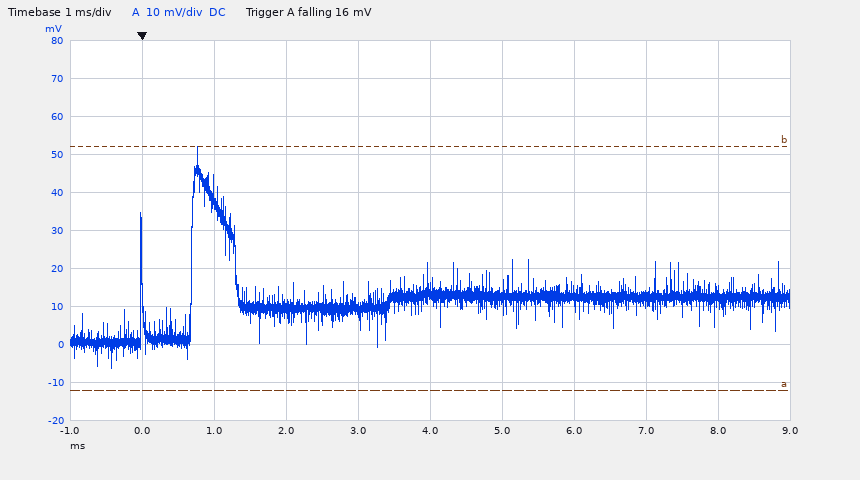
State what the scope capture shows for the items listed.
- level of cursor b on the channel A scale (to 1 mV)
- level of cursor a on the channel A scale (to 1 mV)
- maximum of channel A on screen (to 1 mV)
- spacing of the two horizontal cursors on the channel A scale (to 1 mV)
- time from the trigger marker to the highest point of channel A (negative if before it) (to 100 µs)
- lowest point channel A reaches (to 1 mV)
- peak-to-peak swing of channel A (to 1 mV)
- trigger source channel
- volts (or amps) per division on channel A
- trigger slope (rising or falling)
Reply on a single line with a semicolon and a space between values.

52 mV; -12 mV; 52 mV; 64 mV; +800 µs; -6 mV; 58 mV; channel A; 10 mV; falling
